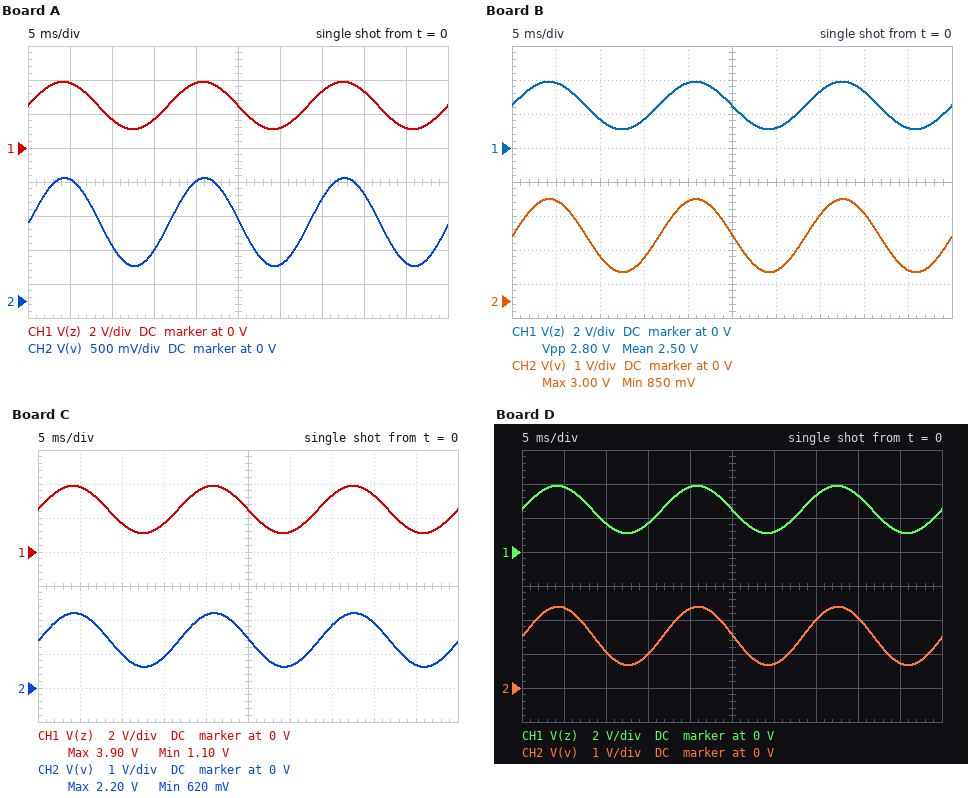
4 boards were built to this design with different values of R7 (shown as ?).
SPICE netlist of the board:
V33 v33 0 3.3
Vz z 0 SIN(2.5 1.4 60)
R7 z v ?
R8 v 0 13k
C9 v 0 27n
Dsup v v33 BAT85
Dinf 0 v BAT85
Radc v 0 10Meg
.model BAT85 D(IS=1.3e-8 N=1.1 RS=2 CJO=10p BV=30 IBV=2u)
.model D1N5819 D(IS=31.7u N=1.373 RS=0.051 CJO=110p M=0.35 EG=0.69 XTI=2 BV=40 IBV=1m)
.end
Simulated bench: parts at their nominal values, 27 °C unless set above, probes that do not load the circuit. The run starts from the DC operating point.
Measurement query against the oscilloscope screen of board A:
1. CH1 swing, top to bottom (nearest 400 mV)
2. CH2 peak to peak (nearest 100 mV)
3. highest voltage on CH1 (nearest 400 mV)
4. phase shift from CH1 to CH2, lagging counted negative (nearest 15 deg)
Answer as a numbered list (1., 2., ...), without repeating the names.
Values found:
1. 2.8 V
2. 1.3 V
3. 4.0 V
4. 0 deg
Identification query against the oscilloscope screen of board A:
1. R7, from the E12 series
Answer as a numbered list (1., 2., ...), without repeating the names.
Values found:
1. 15 kΩ
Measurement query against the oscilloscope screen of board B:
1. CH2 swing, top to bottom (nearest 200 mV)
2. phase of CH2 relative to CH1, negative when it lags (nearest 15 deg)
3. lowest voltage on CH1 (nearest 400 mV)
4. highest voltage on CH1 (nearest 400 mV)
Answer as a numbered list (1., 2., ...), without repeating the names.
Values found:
1. 2.2 V
2. 0 deg
3. 1.2 V
4. 4.0 V
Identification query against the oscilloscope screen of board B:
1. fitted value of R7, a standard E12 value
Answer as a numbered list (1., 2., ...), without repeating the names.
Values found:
1. 3.9 kΩ
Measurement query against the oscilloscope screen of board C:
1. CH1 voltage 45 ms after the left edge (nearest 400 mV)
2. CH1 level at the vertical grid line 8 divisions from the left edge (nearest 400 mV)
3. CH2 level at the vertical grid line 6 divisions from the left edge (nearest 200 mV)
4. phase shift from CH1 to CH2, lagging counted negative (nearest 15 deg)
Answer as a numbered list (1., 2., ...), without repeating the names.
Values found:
1. 1.2 V
2. 3.2 V
3. 600 mV
4. 0 deg
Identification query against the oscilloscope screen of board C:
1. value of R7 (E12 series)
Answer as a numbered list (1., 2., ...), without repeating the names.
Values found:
1. 10 kΩ
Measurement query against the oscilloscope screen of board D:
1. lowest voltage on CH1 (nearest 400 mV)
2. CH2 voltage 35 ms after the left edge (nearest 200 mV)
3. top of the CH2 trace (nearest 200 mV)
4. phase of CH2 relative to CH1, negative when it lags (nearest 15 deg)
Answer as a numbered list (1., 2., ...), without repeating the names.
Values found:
1. 1.2 V
2. 2.0 V
3. 2.4 V
4. 0 deg
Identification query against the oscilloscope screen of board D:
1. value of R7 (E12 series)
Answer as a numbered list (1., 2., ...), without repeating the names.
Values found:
1. 8.2 kΩ
